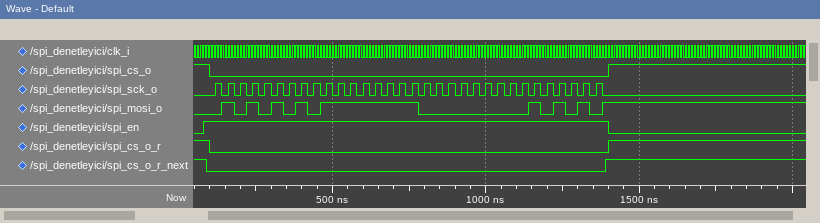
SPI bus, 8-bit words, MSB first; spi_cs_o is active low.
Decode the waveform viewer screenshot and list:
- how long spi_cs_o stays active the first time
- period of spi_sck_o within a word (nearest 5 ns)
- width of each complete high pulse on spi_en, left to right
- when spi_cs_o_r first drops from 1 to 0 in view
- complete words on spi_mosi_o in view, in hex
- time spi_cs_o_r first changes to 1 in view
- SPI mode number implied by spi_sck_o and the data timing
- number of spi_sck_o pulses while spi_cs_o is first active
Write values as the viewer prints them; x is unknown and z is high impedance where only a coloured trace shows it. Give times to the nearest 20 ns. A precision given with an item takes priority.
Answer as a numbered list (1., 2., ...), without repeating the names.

1. 1300 ns
2. 40 ns
3. 1320 ns
4. 100 ns
5. 55, 7F, 80, 2A
6. 1400 ns
7. 0
8. 32
